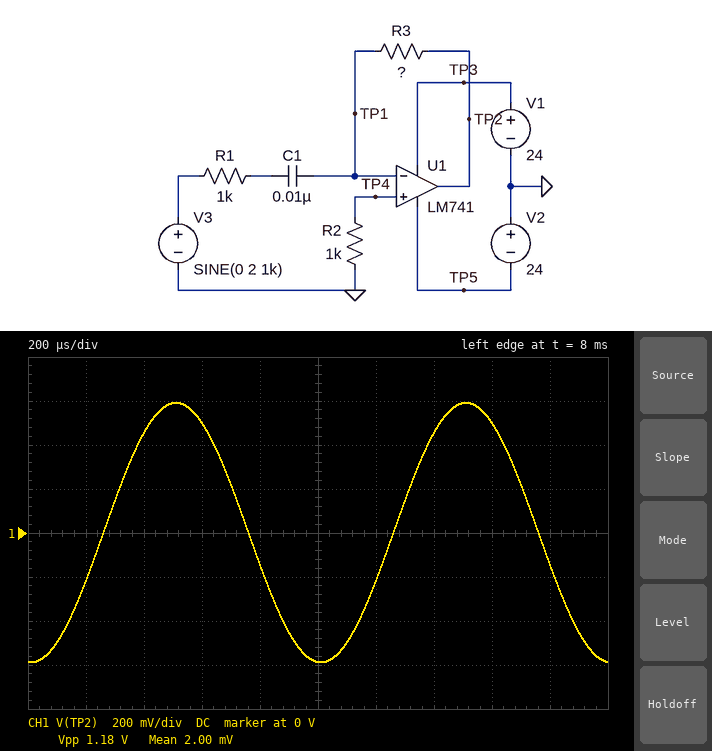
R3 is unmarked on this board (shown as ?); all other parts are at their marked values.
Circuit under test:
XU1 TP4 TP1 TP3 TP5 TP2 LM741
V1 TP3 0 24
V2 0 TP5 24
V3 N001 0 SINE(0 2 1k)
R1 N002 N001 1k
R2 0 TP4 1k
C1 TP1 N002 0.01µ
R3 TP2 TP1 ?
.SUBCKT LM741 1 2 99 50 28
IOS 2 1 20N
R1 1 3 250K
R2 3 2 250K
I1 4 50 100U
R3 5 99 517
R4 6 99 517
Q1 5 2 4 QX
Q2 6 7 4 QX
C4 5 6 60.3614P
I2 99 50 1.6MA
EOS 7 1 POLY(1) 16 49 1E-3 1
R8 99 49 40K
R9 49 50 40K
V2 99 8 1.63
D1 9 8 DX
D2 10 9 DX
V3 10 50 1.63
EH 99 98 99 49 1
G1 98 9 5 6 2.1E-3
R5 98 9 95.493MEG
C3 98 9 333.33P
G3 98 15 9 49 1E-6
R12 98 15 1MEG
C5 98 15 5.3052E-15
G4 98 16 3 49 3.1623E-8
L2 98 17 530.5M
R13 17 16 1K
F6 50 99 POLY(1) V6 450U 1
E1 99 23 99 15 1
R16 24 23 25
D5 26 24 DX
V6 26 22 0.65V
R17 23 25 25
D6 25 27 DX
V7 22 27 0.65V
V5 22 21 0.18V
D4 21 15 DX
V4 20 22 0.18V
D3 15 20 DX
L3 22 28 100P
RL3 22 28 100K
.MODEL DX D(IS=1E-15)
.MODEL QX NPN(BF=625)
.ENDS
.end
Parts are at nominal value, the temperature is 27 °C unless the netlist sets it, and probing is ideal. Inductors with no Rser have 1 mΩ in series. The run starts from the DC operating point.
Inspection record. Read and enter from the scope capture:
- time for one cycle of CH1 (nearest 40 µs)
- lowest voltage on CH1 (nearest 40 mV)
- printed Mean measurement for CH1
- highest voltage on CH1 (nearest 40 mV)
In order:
1.00 ms
-600 mV
2.00 mV
600 mV
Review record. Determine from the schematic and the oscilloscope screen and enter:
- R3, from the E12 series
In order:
4.7 kΩ
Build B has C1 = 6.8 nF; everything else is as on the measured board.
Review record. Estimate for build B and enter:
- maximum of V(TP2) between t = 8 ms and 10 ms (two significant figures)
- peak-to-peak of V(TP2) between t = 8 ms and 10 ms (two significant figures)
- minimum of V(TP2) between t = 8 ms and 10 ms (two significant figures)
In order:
400 mV
800 mV
-400 mV
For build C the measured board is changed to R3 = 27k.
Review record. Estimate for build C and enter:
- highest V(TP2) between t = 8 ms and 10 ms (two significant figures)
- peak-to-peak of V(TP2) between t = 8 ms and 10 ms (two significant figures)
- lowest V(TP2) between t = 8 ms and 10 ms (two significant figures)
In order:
3.4 V
6.8 V
-3.4 V
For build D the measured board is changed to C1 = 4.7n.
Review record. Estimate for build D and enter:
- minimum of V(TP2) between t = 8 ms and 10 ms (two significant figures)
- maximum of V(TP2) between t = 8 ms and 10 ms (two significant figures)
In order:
-280 mV
280 mV
